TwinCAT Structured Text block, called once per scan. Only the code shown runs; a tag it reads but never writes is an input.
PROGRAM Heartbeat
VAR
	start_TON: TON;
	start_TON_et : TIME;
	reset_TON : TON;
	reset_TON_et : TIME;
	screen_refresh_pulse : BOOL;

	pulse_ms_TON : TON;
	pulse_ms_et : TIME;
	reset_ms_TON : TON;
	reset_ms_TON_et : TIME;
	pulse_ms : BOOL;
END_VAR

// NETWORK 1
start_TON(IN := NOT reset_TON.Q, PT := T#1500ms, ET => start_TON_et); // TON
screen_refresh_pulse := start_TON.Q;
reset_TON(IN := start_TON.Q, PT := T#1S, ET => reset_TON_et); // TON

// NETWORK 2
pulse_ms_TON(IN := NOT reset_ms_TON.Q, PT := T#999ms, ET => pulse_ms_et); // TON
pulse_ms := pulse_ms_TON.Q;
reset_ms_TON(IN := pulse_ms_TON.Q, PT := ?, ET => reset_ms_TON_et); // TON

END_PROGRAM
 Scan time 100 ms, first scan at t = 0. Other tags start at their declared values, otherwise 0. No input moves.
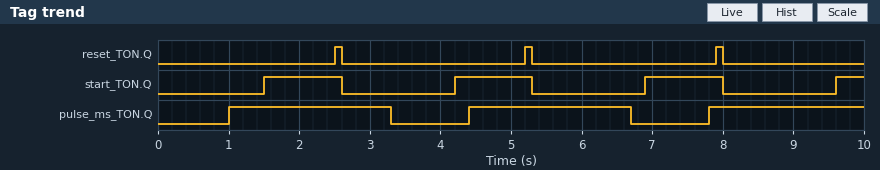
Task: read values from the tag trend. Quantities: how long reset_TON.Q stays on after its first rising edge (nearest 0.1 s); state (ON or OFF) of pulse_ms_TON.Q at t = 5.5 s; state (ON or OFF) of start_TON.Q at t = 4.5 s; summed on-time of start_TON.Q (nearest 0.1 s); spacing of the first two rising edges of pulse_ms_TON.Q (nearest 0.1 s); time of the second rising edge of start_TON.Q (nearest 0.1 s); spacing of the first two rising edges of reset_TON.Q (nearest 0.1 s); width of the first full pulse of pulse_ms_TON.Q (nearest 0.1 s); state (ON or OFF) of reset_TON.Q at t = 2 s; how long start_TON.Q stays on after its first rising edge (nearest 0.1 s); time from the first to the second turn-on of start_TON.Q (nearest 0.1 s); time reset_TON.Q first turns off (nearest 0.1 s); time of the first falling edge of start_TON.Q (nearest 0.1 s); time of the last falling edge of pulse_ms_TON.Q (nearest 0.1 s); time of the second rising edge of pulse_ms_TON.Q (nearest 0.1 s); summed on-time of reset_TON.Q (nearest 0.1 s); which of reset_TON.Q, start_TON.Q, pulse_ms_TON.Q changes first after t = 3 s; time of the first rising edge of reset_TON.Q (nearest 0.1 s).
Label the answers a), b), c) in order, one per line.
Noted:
a) 0.1 s
b) ON
c) ON
d) 3.7 s
e) 3.4 s
f) 4.2 s
g) 2.7 s
h) 2.3 s
i) OFF
j) 1.1 s
k) 2.7 s
l) 2.6 s
m) 2.6 s
n) 6.7 s
o) 4.4 s
p) 0.3 s
q) pulse_ms_TON.Q
r) 2.5 s
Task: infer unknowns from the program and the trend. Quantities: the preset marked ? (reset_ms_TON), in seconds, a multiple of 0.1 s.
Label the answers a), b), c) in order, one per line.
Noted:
a) 2.2 s
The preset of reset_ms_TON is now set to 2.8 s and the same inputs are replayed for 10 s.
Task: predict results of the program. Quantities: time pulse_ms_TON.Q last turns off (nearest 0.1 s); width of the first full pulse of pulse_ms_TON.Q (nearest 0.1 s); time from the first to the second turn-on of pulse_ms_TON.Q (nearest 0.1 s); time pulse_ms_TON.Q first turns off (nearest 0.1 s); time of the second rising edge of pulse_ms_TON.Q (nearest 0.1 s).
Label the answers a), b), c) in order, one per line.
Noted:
a) 7.9 s
b) 2.9 s
c) 4.0 s
d) 3.9 s
e) 5.0 s
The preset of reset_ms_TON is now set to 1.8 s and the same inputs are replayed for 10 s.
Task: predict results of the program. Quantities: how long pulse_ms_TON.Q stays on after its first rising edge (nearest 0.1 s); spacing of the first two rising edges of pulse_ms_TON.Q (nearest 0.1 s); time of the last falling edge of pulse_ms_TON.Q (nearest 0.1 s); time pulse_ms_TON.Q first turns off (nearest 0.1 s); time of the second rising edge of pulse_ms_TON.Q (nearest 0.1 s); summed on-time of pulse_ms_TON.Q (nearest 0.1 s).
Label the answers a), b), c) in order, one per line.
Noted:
a) 1.9 s
b) 3.0 s
c) 8.9 s
d) 2.9 s
e) 4.0 s
f) 5.7 s
